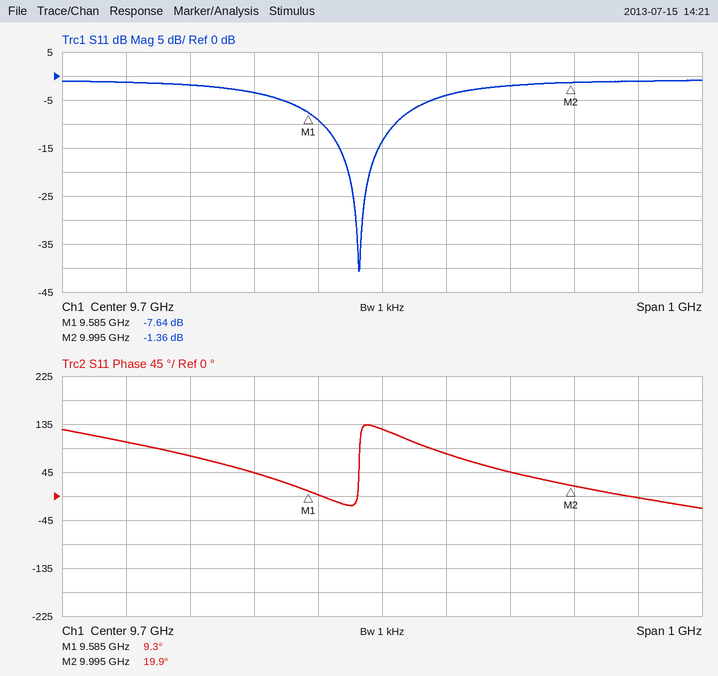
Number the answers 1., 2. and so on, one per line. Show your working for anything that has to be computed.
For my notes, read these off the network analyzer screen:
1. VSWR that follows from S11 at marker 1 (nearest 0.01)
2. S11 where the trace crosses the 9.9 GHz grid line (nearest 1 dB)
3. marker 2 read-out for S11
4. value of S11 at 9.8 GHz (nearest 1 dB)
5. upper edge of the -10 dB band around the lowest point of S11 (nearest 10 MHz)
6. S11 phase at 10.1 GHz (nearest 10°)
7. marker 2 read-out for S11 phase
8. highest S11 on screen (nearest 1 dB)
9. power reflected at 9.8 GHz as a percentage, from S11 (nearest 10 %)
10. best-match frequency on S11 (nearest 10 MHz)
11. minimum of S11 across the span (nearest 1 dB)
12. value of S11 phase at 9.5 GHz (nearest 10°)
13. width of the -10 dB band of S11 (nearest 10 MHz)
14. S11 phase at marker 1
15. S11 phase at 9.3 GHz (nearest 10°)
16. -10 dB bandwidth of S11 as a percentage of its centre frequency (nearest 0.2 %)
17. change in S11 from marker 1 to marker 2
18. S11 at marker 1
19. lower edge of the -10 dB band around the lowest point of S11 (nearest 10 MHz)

1. (1 + 0.4150)/(1 − 0.4150) ≈ 2.42
2. -2 dB
3. -1.36 dB
4. -4 dB
5. 9.72 GHz
6. 0°
7. 19.9°
8. -1 dB
9. 10^(-4/10) ≈ 40 %
10. 9.66 GHz
11. -41 dB
12. 40°
13. 9.72 GHz − 9.61 GHz = 110 MHz
14. 9.3°
15. 100°
16. 110 MHz / 9.665 GHz ≈ 1.14 %, so 1.2 % to the nearest 0.2 %
17. -1.36 − (-7.64) = 6.28 dB
18. -7.64 dB
19. 9.61 GHz
